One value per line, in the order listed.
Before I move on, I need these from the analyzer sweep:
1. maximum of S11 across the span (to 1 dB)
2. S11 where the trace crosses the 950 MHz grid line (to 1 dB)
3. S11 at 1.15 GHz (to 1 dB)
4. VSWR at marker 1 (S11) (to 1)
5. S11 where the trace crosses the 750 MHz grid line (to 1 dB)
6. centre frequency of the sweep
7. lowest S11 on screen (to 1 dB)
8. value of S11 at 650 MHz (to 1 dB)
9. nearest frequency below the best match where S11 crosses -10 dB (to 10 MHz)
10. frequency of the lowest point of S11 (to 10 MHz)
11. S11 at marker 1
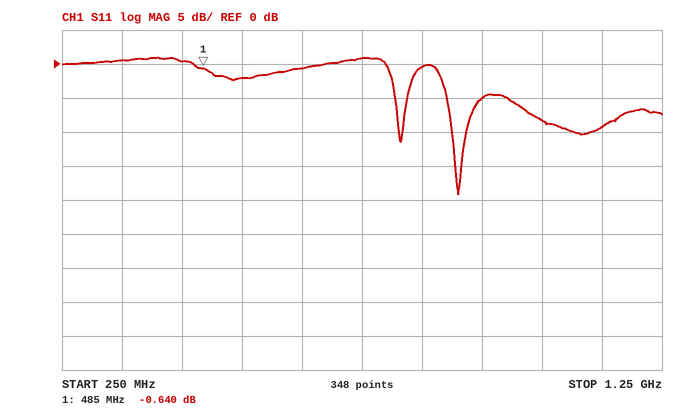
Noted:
1 dB
-5 dB
-9 dB
27
1 dB
750 MHz
-19 dB
-1 dB
900 MHz
910 MHz
-0.640 dB
